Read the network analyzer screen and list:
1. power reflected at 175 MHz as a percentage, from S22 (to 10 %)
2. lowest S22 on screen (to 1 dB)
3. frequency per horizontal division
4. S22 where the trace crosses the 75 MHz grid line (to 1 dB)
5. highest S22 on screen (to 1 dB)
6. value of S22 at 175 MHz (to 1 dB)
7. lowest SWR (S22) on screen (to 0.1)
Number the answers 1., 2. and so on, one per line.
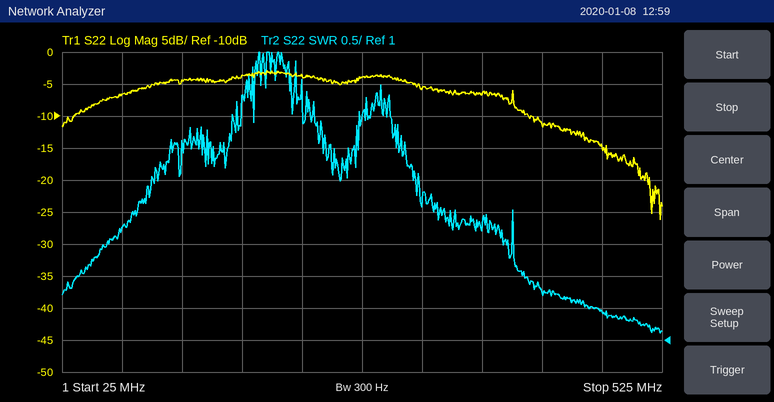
1. 40 %
2. -26 dB
3. 50 MHz
4. -7 dB
5. -3 dB
6. -4 dB
7. 1.1
